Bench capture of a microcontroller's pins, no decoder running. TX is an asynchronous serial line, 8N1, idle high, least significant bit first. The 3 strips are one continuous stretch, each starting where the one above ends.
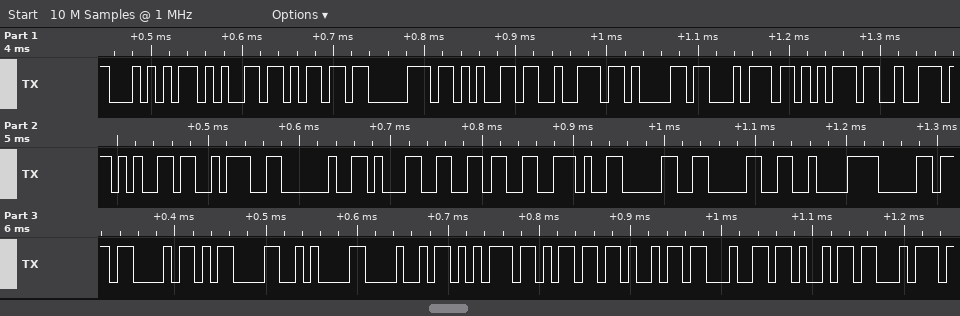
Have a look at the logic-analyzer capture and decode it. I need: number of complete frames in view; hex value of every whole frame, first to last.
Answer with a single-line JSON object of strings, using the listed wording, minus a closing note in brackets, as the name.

{"number of complete frames in view": "30", "hex value of every whole frame, first to last": "54 65 6D 70 65 72 61 74 75 72 65 3A 20 31 36 2E 30 30 C2 B0 43 0D 0A 48 75 6D 69 64 69 74"}
